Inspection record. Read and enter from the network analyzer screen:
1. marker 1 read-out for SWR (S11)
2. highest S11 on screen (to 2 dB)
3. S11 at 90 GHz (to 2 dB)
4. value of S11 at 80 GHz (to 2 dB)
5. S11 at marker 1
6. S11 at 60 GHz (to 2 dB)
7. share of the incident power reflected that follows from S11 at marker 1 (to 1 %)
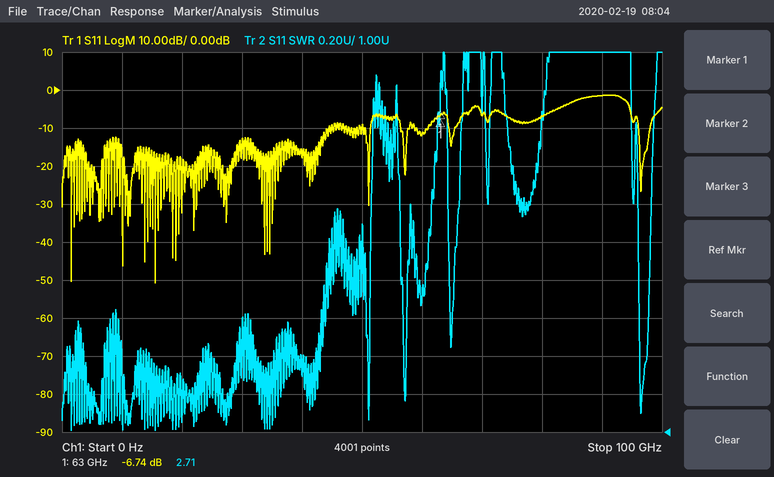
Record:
2.71
-2 dB
-2 dB
-6 dB
-6.74 dB
-12 dB
21 %
